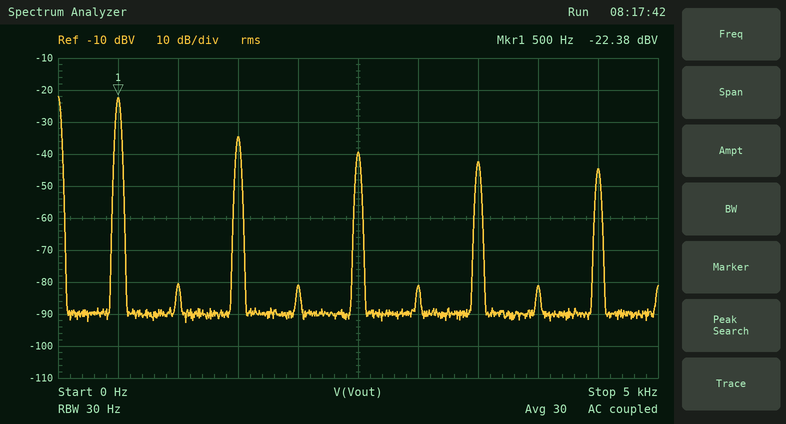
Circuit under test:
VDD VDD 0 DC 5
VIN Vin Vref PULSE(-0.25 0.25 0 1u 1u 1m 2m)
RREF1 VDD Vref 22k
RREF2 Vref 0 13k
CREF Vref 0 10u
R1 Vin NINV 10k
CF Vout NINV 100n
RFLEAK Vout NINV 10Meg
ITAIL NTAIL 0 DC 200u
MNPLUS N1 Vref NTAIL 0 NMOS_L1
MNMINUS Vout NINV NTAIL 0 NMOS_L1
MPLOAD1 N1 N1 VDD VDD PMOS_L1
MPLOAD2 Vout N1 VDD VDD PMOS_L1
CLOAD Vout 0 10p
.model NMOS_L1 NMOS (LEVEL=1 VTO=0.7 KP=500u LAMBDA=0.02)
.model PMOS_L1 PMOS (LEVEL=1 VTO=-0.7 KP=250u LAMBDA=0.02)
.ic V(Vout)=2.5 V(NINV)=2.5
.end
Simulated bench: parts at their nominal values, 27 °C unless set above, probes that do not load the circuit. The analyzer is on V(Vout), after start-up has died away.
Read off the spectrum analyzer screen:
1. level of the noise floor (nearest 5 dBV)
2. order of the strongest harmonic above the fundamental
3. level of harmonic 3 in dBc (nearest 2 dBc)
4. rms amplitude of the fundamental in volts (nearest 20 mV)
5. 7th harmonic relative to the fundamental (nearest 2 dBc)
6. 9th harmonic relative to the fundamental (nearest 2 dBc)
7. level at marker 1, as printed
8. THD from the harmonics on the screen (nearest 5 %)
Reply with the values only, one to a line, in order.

-90 dBV
3
-12 dBc
80 mV
-20 dBc
-22 dBc
-22.38 dBV
30 %
